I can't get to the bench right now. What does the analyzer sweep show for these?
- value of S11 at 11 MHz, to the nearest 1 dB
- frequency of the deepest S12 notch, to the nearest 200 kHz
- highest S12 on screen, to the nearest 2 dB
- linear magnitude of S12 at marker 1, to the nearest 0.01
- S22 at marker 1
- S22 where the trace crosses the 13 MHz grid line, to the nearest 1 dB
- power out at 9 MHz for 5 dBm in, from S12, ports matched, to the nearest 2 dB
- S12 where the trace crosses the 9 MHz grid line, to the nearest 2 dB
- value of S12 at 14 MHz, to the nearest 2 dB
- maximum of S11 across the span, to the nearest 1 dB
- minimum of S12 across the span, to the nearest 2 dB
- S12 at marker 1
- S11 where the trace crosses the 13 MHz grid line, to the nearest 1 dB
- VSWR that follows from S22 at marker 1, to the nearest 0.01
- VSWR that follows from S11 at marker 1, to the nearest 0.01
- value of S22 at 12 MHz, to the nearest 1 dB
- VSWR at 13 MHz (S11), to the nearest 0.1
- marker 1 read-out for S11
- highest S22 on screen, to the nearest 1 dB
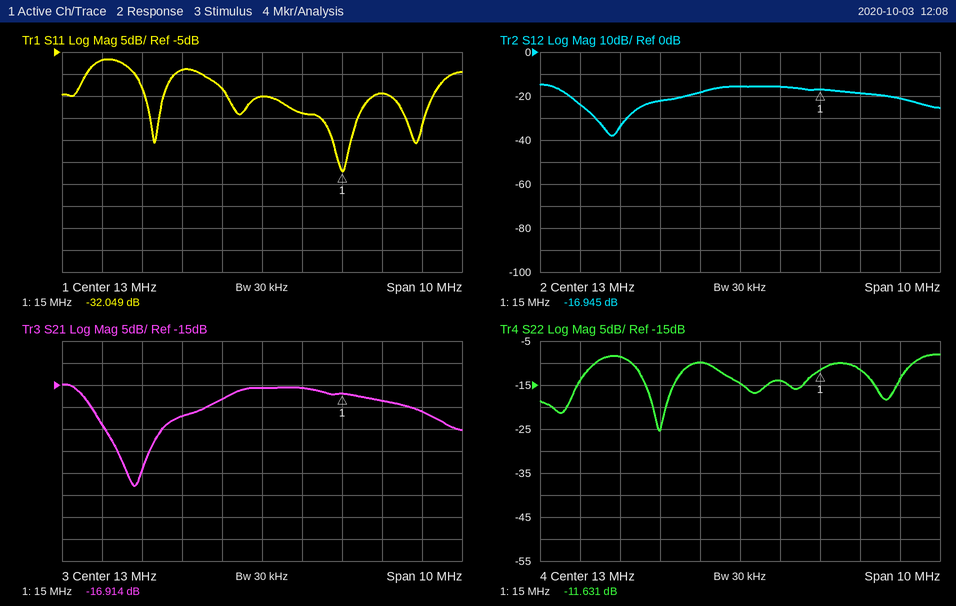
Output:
-9 dB
9.8 MHz
-14 dB
0.14
-11.631 dB
-15 dB
-18 dBm
-24 dB
-16 dB
-7 dB
-38 dB
-16.945 dB
-15 dB
1.71
1.05
-10 dB
1.4
-32.049 dB
-8 dB
